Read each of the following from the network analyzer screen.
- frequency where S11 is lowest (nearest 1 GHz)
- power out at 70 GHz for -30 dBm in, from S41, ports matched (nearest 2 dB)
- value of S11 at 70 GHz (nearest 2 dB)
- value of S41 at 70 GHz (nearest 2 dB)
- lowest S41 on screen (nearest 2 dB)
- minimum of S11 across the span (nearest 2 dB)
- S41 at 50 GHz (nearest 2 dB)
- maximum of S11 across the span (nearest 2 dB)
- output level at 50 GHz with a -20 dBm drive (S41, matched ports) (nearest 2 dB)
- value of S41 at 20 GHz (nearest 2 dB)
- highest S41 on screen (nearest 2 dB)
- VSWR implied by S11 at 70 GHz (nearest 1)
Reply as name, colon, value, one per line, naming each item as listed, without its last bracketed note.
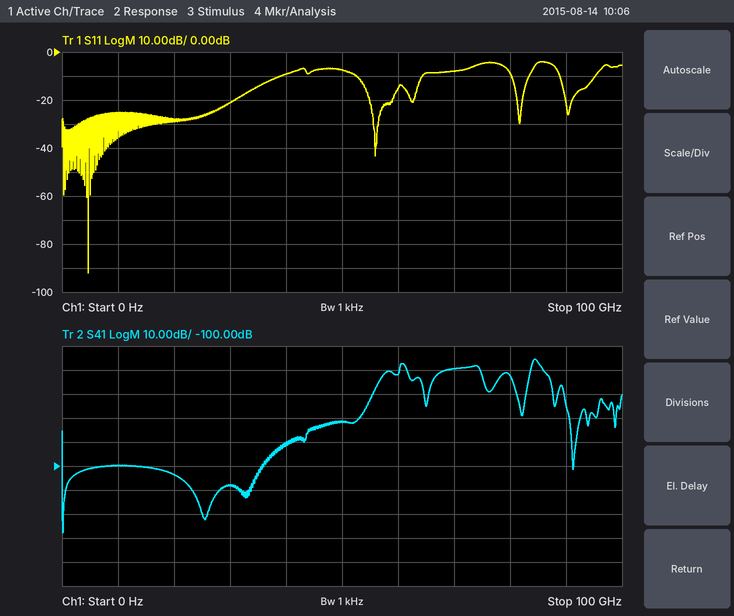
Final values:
frequency where S11 is lowest: 5 GHz
power out at 70 GHz for -30 dBm in, from S41, ports matched: -90 dBm
value of S11 at 70 GHz: -8 dB
value of S41 at 70 GHz: -60 dB
lowest S41 on screen: -128 dB
minimum of S11 across the span: -92 dB
S41 at 50 GHz: -82 dB
maximum of S11 across the span: -4 dB
output level at 50 GHz with a -20 dBm drive (S41, matched ports): -102 dBm
value of S41 at 20 GHz: -104 dB
highest S41 on screen: -56 dB
VSWR implied by S11 at 70 GHz: 2
